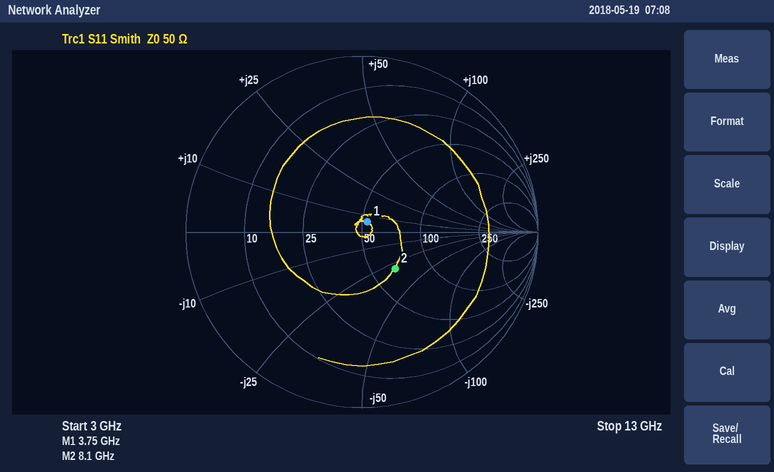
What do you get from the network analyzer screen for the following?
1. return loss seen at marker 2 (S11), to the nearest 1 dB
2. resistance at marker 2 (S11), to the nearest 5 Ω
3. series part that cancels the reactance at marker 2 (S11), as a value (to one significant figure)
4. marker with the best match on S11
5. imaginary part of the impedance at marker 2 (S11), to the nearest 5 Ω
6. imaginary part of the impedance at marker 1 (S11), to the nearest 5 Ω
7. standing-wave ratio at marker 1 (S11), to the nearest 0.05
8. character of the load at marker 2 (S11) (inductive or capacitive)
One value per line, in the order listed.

11 dB
65 Ω
600 pH
marker 1
-30 Ω
+5 Ω
1.15
capacitive
